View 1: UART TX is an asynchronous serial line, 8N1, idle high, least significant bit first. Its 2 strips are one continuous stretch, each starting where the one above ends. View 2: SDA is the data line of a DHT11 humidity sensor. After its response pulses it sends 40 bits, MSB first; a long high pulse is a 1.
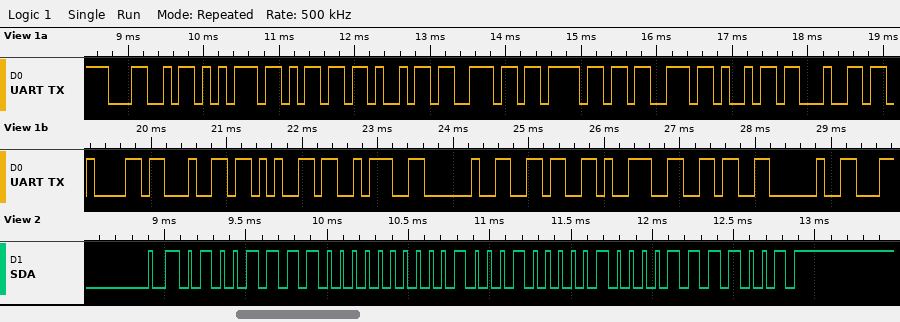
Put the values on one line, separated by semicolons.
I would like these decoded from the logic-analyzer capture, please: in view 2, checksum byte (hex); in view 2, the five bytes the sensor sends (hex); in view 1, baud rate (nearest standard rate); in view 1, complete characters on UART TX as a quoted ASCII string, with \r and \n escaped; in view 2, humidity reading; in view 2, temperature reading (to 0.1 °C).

0x79; 4F 00 22 08 79; 9600 baud; "Luminosidade: 696 "; 79 %; 34.8 °C
